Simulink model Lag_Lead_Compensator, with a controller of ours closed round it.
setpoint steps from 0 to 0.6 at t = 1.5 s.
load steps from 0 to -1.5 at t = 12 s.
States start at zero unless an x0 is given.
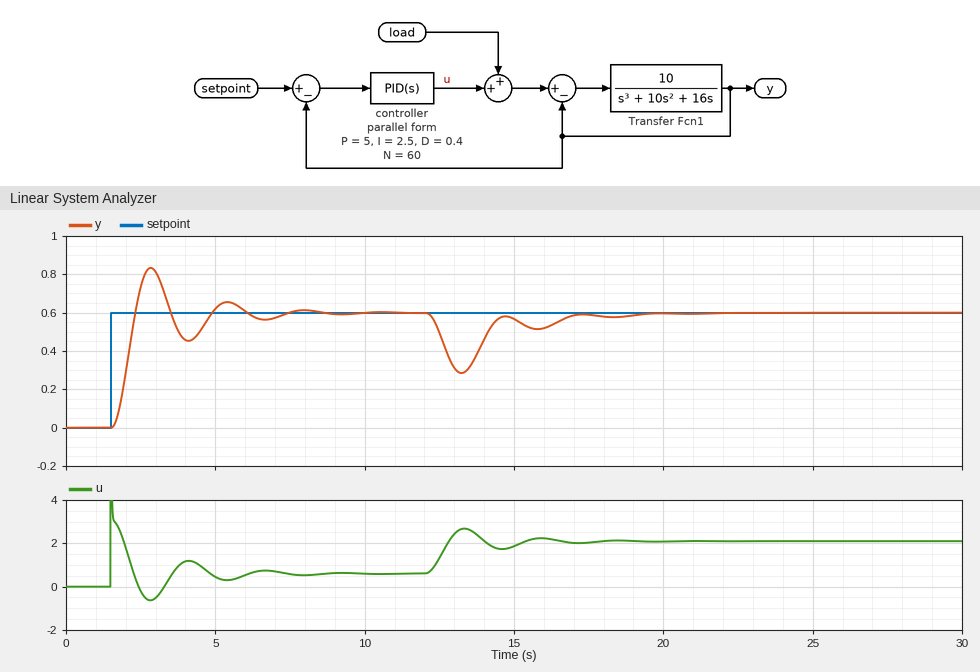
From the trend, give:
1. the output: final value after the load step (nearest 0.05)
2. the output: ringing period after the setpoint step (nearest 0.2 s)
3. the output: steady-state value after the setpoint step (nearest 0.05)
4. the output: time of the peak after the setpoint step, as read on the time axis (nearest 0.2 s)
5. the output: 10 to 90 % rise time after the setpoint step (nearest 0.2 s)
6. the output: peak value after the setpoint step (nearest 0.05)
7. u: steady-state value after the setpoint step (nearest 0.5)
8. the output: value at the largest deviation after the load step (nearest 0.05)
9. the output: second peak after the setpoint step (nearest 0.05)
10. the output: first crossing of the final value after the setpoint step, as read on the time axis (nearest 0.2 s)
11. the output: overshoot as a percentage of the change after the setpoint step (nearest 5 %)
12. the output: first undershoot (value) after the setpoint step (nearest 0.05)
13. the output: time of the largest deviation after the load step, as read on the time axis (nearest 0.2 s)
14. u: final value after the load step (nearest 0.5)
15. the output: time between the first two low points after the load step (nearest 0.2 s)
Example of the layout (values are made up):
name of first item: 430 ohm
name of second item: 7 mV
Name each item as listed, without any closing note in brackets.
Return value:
the output: final value after the load step: 0.60
the output: ringing period after the setpoint step: 2.6 s
the output: steady-state value after the setpoint step: 0.60
the output: time of the peak after the setpoint step, as read on the time axis: 2.8 s
the output: 10 to 90 % rise time after the setpoint step: 0.6 s
the output: peak value after the setpoint step: 0.85
u: steady-state value after the setpoint step: 0.5
the output: value at the largest deviation after the load step: 0.30
the output: second peak after the setpoint step: 0.65
the output: first crossing of the final value after the setpoint step, as read on the time axis: 2.4 s
the output: overshoot as a percentage of the change after the setpoint step: 40 %
the output: first undershoot (value) after the setpoint step: 0.45
the output: time of the largest deviation after the load step, as read on the time axis: 13.2 s
u: final value after the load step: 2.0
the output: time between the first two low points after the load step: 2.6 s
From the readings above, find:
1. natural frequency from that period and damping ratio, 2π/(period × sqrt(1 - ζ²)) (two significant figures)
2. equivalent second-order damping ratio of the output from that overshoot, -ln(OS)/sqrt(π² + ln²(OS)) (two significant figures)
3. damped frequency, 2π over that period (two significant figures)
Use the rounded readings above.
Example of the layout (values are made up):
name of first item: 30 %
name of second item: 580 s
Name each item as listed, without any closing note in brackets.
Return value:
natural frequency from that period and damping ratio, 2π/(period × sqrt(1 - ζ²)): 2.5 rad/s
equivalent second-order damping ratio of the output from that overshoot, -ln(OS)/sqrt(π² + ln²(OS)): 0.28
damped frequency, 2π over that period: 2.4 rad/s
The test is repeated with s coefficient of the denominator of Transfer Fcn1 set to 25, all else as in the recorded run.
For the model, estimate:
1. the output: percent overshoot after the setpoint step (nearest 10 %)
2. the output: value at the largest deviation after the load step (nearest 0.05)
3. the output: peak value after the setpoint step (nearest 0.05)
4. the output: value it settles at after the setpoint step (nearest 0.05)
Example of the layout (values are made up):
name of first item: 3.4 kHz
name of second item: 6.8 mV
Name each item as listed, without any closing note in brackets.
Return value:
the output: percent overshoot after the setpoint step: 20 %
the output: value at the largest deviation after the load step: 0.35
the output: peak value after the setpoint step: 0.70
the output: value it settles at after the setpoint step: 0.60
